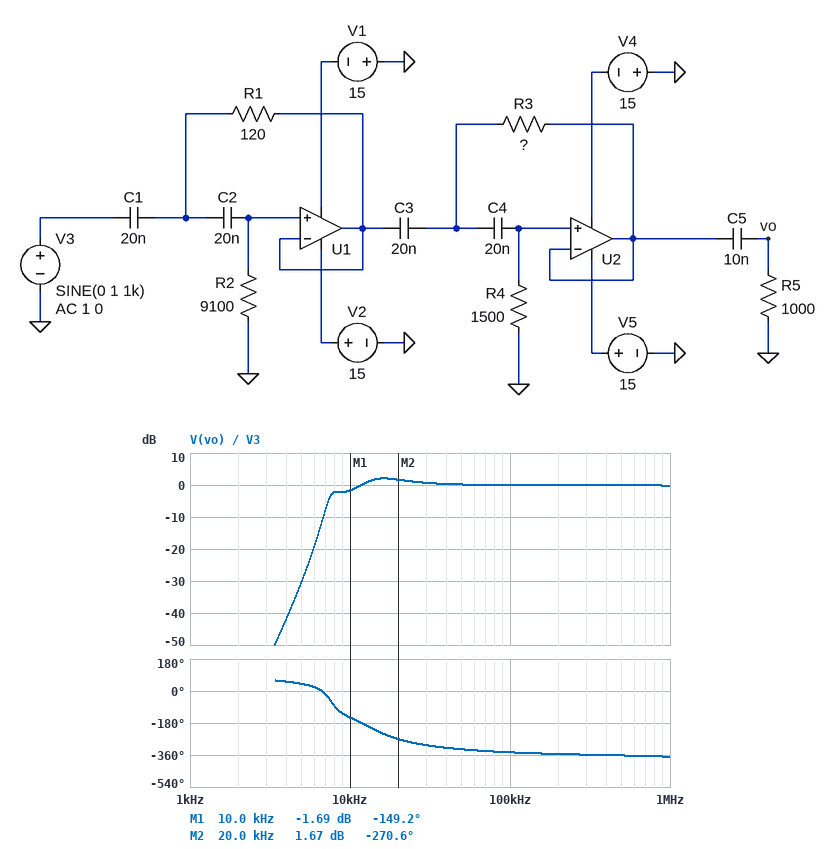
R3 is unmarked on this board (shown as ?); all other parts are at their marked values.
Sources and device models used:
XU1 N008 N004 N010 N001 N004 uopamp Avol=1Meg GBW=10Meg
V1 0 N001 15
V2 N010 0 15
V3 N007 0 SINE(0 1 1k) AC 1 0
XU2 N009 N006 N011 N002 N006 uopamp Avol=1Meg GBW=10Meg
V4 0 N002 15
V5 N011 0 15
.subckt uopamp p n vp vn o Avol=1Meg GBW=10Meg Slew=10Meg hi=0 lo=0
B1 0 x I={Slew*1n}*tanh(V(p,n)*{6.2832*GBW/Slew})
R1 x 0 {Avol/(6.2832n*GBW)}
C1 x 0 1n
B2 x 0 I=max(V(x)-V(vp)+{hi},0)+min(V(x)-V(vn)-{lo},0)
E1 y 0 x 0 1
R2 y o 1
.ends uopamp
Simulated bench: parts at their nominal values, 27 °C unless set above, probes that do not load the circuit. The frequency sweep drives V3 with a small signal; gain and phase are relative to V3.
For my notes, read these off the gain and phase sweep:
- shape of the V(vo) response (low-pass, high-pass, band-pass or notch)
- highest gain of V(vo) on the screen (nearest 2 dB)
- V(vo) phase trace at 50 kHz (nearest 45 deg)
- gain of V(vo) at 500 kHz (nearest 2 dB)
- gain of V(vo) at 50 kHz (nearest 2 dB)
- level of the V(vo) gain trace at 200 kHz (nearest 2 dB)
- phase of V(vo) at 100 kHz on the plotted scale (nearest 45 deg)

high-pass
2 dB
-315 deg
0 dB
0 dB
0 dB
-360 deg
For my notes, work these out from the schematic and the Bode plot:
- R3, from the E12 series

220 Ω
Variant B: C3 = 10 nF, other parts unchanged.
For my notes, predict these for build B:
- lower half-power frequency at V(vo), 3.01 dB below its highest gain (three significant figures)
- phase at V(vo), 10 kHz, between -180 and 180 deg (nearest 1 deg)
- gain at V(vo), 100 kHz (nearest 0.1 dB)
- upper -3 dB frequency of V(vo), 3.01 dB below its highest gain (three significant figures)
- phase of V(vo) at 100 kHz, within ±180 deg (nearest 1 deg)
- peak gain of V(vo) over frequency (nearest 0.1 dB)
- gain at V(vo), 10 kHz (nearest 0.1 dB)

16.6 kHz
-129 deg
0 dB
3.66 MHz
18 deg
1.8 dB
-9.0 dB
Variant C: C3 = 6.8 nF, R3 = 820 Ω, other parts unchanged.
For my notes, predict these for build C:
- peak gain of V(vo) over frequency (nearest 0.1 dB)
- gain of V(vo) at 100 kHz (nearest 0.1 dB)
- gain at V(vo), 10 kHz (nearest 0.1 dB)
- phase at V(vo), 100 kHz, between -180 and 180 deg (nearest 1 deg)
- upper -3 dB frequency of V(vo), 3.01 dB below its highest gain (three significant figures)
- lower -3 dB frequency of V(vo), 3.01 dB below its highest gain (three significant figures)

-0.1 dB
-0.2 dB
-5.4 dB
21 deg
6.46 MHz
17.8 kHz
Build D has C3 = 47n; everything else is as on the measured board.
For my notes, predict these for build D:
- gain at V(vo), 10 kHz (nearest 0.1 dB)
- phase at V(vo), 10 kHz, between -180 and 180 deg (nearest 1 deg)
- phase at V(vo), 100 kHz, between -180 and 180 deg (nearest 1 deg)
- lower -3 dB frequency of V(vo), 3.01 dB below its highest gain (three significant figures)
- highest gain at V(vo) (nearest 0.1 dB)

3.4 dB
156 deg
13 deg
7.24 kHz
5.6 dB
